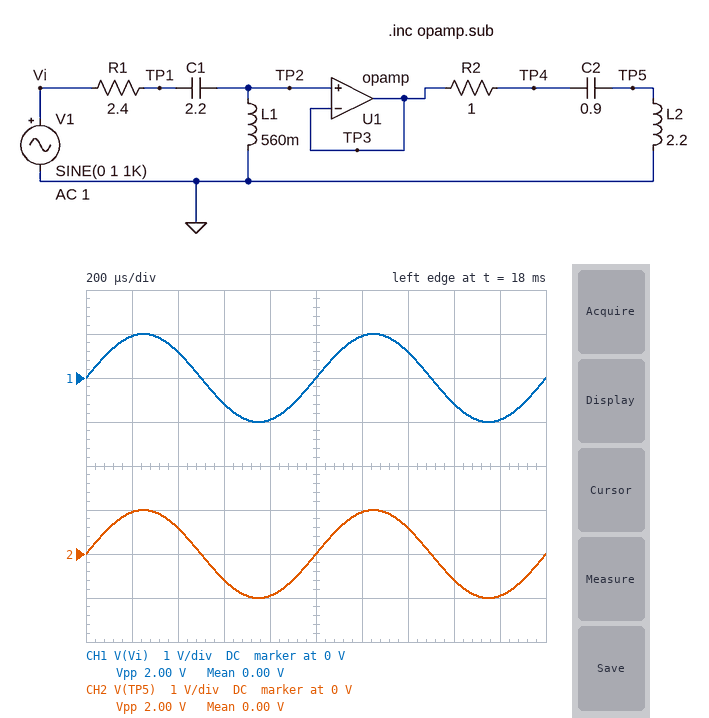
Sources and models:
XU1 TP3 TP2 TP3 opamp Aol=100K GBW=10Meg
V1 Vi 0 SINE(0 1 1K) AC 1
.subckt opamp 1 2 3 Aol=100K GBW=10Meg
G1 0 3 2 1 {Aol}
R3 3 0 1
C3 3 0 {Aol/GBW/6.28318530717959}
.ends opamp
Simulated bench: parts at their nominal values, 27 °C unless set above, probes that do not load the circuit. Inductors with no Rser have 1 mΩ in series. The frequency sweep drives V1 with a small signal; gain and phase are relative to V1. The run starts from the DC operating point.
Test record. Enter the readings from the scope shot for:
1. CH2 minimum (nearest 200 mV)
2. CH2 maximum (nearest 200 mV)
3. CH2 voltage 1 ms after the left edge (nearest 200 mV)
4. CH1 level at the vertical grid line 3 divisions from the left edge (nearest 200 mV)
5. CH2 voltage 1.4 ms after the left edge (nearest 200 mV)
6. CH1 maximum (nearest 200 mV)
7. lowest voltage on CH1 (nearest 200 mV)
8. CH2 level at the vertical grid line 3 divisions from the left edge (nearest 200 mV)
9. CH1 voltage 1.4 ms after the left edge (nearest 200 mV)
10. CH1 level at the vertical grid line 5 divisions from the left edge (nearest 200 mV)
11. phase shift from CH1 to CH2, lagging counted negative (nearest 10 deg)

-1.0 V
1.0 V
0 V
-600 mV
600 mV
1.0 V
-1.0 V
-600 mV
600 mV
0 V
0 deg
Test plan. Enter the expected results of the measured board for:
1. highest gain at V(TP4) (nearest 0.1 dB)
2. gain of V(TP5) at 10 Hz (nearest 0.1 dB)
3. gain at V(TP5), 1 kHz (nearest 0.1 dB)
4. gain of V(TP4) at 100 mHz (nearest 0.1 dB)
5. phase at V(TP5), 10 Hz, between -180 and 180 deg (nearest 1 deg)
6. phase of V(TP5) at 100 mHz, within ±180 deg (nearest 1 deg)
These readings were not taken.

0 dB
0 dB
0 dB
-25.7 dB
4 deg
-150 deg
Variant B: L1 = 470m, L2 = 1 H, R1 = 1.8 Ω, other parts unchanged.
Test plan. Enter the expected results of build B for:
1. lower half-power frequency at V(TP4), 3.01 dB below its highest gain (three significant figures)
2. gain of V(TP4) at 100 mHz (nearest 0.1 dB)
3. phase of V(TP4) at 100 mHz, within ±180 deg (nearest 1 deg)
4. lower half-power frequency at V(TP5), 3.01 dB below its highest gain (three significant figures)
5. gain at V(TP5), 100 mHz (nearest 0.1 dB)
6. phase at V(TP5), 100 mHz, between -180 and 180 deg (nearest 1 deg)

616 mHz
-18.4 dB
62 deg
513 mHz
-23.6 dB
-118 deg
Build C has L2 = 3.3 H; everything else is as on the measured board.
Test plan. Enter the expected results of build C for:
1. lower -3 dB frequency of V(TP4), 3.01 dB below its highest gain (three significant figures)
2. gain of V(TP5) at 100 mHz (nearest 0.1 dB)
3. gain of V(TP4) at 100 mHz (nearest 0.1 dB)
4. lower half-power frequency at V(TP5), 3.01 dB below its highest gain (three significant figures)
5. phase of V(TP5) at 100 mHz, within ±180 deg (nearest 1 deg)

656 mHz
-10.8 dB
-27.5 dB
629 mHz
172 deg
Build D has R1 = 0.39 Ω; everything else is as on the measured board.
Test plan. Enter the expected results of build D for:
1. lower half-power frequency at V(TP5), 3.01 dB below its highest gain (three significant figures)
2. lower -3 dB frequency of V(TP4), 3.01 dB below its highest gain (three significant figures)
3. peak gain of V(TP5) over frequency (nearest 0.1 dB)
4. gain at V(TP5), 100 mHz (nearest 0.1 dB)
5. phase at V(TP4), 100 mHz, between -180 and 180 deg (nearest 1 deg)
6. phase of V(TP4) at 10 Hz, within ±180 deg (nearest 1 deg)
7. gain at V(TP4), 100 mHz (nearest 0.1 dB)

116 mHz
147 mHz
6.3 dB
-1.5 dB
65 deg
1 deg
-12.6 dB
